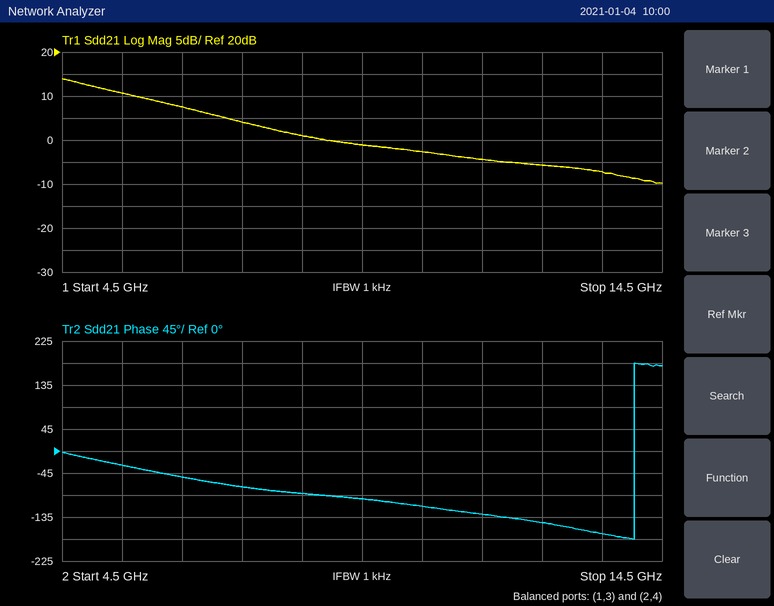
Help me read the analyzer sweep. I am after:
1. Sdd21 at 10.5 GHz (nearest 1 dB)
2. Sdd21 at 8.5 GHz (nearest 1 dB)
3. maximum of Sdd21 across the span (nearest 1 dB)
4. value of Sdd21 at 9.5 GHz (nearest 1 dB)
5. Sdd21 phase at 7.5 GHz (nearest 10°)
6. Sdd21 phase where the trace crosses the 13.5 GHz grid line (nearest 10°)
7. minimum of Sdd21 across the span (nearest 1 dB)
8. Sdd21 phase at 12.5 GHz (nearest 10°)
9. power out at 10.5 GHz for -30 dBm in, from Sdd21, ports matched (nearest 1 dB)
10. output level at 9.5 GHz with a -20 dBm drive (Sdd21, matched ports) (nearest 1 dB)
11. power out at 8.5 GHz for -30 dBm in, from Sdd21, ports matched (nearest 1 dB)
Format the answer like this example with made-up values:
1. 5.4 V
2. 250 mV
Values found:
1. -3 dB
2. 1 dB
3. 14 dB
4. -1 dB
5. -70°
6. -170°
7. -10 dB
8. -150°
9. -33 dBm
10. -21 dBm
11. -29 dBm
